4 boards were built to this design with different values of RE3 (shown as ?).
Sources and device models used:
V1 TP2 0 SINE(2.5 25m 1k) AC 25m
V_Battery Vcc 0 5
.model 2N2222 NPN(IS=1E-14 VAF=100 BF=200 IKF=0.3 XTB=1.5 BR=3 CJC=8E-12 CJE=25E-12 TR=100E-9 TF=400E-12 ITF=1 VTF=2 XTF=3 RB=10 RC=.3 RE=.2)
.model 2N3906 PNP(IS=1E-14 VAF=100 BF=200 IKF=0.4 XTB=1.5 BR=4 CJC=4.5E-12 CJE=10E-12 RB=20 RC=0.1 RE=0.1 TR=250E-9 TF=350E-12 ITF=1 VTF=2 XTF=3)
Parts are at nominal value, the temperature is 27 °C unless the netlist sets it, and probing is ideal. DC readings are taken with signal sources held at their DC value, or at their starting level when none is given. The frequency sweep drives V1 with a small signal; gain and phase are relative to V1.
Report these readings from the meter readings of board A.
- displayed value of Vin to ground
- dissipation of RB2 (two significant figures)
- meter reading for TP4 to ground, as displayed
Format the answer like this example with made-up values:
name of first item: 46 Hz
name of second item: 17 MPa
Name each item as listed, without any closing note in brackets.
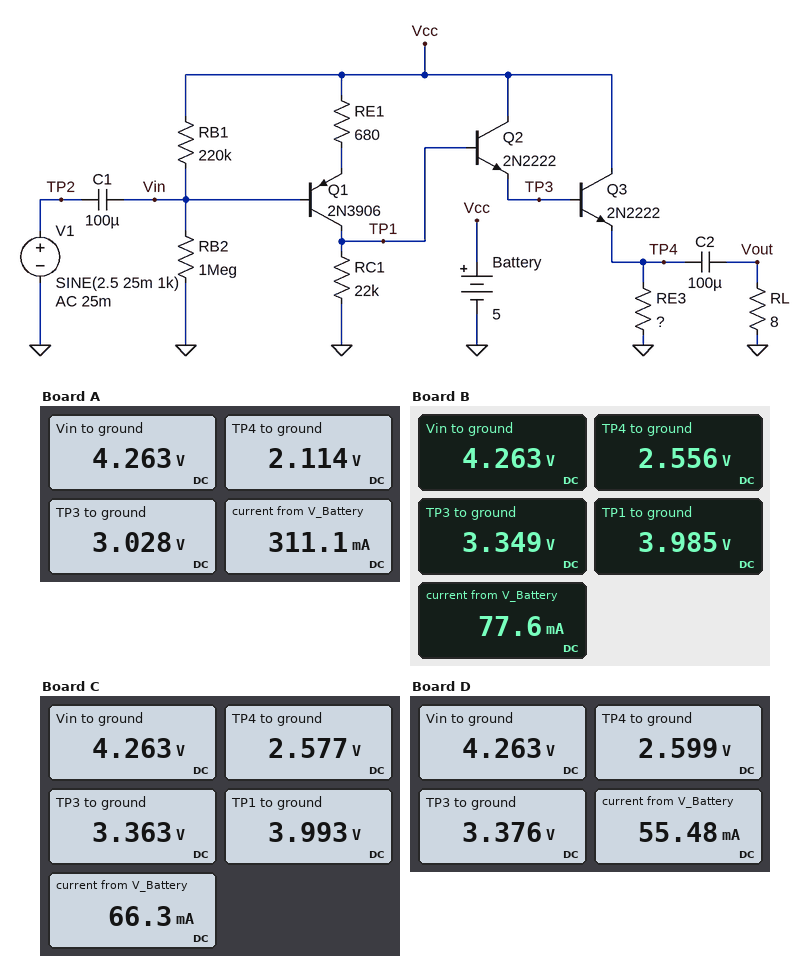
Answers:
displayed value of Vin to ground: 4.263 V
dissipation of RB2: 18 µW
meter reading for TP4 to ground, as displayed: 2.114 V
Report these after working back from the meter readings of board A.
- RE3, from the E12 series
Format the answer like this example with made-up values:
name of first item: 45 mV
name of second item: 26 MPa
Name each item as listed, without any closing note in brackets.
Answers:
RE3, from the E12 series: 6.8 Ω
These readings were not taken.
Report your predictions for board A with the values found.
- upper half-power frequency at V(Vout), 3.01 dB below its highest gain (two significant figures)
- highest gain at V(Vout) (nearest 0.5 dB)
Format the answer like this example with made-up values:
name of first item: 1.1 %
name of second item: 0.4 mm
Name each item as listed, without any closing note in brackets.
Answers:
upper half-power frequency at V(Vout), 3.01 dB below its highest gain: 810 kHz
highest gain at V(Vout): 24.5 dB
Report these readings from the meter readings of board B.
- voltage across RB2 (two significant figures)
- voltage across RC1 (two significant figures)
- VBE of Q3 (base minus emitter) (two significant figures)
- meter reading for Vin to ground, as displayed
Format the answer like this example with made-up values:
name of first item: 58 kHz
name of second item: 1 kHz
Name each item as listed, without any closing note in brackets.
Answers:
voltage across RB2: 4.3 V
voltage across RC1: 4.0 V
VBE of Q3 (base minus emitter): 790 mV
meter reading for Vin to ground, as displayed: 4.263 V
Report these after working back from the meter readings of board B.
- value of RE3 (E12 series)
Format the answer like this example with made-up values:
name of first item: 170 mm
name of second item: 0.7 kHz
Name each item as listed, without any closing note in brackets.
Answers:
value of RE3: 33 Ω
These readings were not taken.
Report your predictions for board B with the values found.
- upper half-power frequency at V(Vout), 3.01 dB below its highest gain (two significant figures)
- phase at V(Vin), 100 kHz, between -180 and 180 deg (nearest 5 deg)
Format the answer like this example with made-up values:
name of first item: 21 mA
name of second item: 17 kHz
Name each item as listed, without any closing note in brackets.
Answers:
upper half-power frequency at V(Vout), 3.01 dB below its highest gain: 650 kHz
phase at V(Vin), 100 kHz, between -180 and 180 deg: 0 deg
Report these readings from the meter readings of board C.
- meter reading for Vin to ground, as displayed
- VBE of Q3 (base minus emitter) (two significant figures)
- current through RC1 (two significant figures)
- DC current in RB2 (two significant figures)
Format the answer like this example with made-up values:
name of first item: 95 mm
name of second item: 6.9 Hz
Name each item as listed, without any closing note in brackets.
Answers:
meter reading for Vin to ground, as displayed: 4.263 V
VBE of Q3 (base minus emitter): 790 mV
current through RC1: 180 µA
DC current in RB2: 4.3 µA
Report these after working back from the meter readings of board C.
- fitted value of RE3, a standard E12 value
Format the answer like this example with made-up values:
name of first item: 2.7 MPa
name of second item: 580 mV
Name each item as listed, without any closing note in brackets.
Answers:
fitted value of RE3, a standard E12 value: 39 Ω
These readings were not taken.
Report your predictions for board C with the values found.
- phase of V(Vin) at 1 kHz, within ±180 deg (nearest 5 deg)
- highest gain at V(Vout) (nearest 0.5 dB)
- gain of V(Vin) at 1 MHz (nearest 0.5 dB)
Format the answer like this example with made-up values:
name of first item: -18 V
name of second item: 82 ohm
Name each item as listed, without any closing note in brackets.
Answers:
phase of V(Vin) at 1 kHz, within ±180 deg: 0 deg
highest gain at V(Vout): 26.0 dB
gain of V(Vin) at 1 MHz: 0 dB
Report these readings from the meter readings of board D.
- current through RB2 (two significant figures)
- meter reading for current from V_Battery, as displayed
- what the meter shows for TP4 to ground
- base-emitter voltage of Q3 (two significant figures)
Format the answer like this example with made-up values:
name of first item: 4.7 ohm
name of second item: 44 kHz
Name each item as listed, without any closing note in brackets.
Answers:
current through RB2: 4.3 µA
meter reading for current from V_Battery, as displayed: 55.48 mA
what the meter shows for TP4 to ground: 2.599 V
base-emitter voltage of Q3: 780 mV
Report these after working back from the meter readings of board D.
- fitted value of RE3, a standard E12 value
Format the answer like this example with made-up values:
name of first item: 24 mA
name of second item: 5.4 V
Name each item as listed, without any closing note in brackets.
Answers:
fitted value of RE3, a standard E12 value: 47 Ω
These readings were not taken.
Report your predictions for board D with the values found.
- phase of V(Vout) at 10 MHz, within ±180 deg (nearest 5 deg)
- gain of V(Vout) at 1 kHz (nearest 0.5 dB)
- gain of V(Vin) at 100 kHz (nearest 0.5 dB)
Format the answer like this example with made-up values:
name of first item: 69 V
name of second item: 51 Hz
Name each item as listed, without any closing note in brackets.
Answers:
phase of V(Vout) at 10 MHz, within ±180 deg: 30 deg
gain of V(Vout) at 1 kHz: 26.0 dB
gain of V(Vin) at 100 kHz: 0 dB
